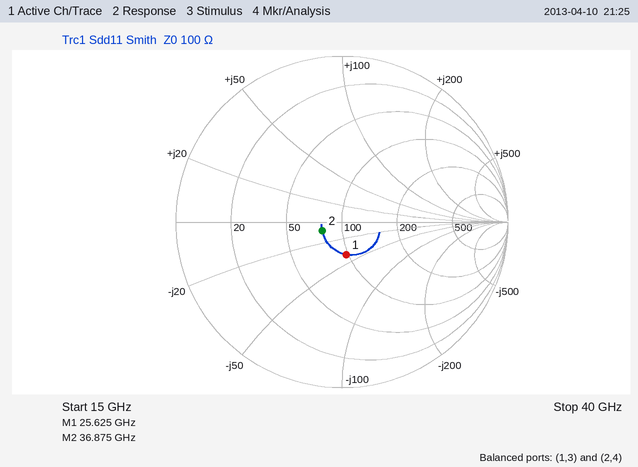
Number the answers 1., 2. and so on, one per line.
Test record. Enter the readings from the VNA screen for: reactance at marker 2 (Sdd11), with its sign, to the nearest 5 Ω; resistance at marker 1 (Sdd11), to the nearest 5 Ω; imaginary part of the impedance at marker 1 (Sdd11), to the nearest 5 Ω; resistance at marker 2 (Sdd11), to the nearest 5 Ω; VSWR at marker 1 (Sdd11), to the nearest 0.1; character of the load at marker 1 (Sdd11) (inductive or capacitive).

1. -10 Ω
2. 95 Ω
3. -40 Ω
4. 80 Ω
5. 1.5
6. capacitive
